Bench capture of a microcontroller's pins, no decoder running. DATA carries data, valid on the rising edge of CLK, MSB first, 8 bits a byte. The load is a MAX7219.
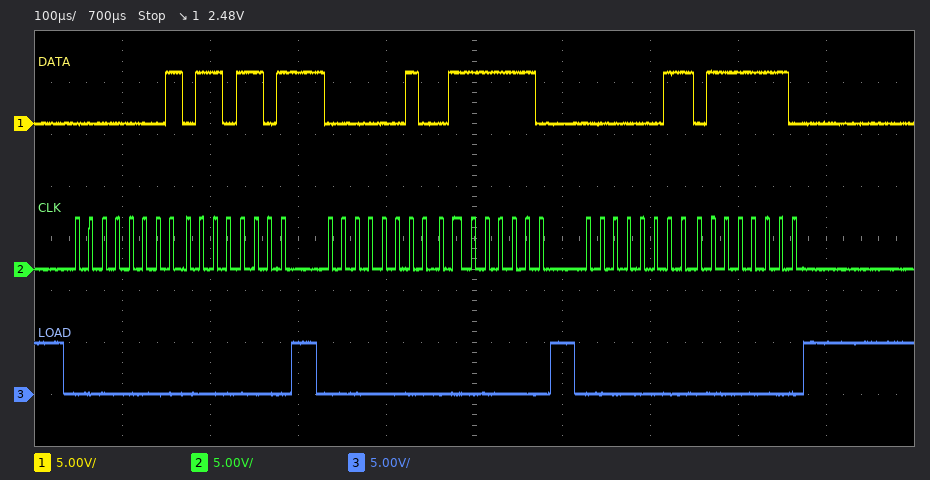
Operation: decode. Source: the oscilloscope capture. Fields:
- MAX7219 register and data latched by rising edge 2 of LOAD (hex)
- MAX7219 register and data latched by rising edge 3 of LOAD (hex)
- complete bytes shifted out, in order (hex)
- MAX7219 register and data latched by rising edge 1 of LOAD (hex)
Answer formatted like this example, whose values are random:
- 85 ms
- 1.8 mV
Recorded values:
- register 0x2, data 0x7E
- register 0x3, data 0x7E
- 0x01 0x6D 0x02 0x7E 0x03 0x7E
- register 0x1, data 0x6D
